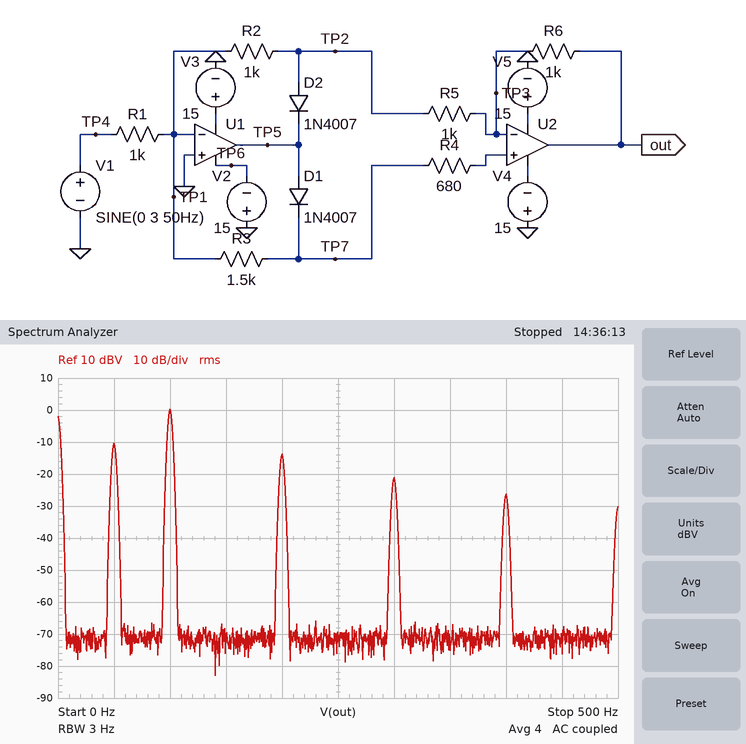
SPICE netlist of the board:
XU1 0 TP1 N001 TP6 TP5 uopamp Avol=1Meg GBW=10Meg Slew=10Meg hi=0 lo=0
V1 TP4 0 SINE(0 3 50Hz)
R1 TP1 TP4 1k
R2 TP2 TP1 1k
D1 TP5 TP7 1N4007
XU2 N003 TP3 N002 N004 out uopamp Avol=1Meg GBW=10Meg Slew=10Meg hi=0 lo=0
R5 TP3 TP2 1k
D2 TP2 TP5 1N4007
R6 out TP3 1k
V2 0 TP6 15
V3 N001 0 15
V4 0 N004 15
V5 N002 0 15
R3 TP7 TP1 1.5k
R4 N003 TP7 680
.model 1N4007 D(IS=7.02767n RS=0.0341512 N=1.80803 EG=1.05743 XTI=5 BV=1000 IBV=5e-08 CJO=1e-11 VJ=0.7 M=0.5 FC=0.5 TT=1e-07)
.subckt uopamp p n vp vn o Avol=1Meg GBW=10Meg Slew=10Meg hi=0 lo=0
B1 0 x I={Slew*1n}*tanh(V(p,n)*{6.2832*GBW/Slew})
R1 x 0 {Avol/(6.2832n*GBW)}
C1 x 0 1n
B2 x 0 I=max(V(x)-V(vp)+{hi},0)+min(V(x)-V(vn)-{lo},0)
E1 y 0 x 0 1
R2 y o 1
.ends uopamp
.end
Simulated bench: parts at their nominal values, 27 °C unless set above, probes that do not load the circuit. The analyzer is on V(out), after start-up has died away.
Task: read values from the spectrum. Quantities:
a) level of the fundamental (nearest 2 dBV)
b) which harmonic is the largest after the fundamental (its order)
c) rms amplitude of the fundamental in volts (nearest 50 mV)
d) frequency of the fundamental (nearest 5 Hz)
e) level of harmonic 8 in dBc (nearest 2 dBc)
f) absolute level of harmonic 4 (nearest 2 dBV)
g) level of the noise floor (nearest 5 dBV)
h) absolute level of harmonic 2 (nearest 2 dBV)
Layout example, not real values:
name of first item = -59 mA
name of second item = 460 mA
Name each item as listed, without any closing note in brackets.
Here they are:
level of the fundamental = -10 dBV
which harmonic is the largest after the fundamental = 2
rms amplitude of the fundamental in volts = 300 mV
frequency of the fundamental = 50 Hz
level of harmonic 8 in dBc = -16 dBc
absolute level of harmonic 4 = -14 dBV
level of the noise floor = -70 dBV
absolute level of harmonic 2 = 0 dBV
